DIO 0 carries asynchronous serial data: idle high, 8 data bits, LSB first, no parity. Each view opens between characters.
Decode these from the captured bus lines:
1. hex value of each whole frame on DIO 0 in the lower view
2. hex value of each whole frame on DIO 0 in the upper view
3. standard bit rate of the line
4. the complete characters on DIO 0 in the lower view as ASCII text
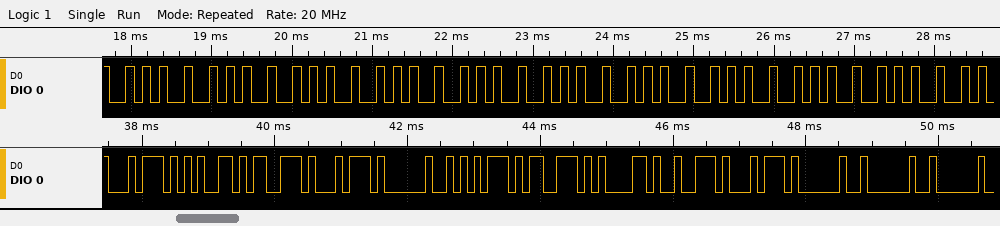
74, 65, 73, 74, 20, 75, 73, 61, 72, 74, 20, 20
2A, 2A, 2A, 2A, 2A, 2A, 2A, 2A, 2A, 2A
9600 baud
"test usart  "
